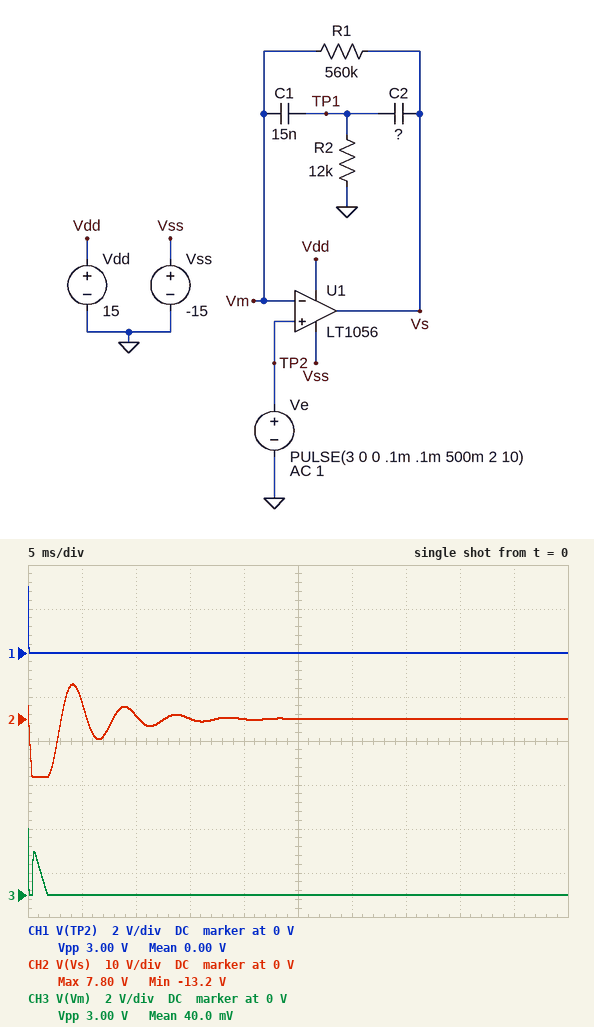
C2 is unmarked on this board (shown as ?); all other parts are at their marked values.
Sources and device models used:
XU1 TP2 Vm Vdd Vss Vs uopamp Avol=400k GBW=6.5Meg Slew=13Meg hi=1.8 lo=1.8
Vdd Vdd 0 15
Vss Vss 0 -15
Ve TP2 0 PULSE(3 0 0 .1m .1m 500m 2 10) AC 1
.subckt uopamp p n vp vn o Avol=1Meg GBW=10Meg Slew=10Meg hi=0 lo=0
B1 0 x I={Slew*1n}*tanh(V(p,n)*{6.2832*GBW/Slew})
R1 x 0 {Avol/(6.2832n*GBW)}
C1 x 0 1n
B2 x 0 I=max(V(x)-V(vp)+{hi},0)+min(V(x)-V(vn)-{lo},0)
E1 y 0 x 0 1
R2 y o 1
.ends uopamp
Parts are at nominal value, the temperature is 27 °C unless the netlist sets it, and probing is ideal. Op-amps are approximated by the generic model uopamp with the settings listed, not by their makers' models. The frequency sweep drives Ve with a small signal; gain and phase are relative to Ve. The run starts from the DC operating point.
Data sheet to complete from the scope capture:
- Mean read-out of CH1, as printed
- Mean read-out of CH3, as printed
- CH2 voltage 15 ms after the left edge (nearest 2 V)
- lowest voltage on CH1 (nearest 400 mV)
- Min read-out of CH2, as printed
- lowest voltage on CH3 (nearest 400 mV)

0.00 V
40.0 mV
0 V
0 V
-13.2 V
0 V
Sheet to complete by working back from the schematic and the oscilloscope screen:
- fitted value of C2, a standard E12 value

5.6 nF
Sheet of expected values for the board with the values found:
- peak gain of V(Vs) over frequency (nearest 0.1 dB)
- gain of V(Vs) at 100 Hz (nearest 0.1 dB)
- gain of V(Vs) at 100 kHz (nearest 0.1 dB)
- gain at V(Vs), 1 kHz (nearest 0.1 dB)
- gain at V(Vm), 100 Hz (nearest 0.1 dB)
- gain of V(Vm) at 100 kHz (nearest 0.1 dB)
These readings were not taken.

30.9 dB
16.8 dB
0 dB
8.7 dB
0 dB
0 dB
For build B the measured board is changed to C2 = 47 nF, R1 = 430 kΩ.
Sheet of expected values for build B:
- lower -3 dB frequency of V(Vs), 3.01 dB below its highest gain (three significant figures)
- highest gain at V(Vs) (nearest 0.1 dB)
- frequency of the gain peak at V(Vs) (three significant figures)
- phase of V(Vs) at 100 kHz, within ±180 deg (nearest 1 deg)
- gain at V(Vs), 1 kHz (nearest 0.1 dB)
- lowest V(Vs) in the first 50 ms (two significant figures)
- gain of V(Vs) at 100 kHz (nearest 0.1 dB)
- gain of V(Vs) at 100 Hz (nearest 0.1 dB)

68.6 Hz
19.7 dB
83.4 Hz
-1 deg
0.4 dB
-7.7 V
0 dB
17.0 dB
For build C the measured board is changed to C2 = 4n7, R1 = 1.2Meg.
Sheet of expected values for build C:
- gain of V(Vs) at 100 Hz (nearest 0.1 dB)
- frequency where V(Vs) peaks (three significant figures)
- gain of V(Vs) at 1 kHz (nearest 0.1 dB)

25.4 dB
158 Hz
9.8 dB
